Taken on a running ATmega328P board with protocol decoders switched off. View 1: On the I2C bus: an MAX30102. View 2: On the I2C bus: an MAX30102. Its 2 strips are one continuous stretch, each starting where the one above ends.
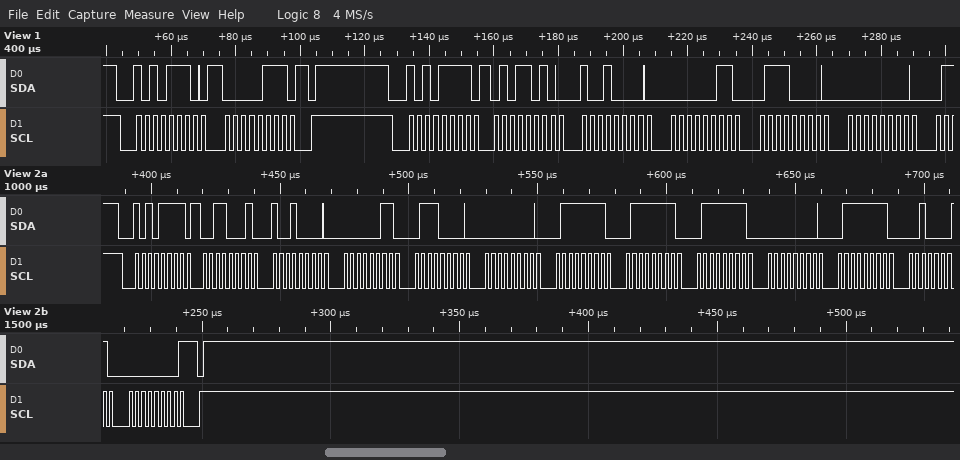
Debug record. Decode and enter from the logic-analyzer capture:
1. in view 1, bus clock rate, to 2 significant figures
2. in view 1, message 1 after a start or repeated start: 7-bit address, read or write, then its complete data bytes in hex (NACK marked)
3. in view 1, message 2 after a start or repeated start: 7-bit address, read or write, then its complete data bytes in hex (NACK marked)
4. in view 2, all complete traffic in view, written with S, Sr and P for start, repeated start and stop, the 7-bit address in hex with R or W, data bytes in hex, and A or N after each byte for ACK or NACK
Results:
400 kHz
0x57 write: 07
0x57 read: 5A 90 03 70 00
S 57R A 31 A 90 A 03 A 70 A 00 A 7F A 7F A 7F A 00 A 7F A 21 A 00 N P
